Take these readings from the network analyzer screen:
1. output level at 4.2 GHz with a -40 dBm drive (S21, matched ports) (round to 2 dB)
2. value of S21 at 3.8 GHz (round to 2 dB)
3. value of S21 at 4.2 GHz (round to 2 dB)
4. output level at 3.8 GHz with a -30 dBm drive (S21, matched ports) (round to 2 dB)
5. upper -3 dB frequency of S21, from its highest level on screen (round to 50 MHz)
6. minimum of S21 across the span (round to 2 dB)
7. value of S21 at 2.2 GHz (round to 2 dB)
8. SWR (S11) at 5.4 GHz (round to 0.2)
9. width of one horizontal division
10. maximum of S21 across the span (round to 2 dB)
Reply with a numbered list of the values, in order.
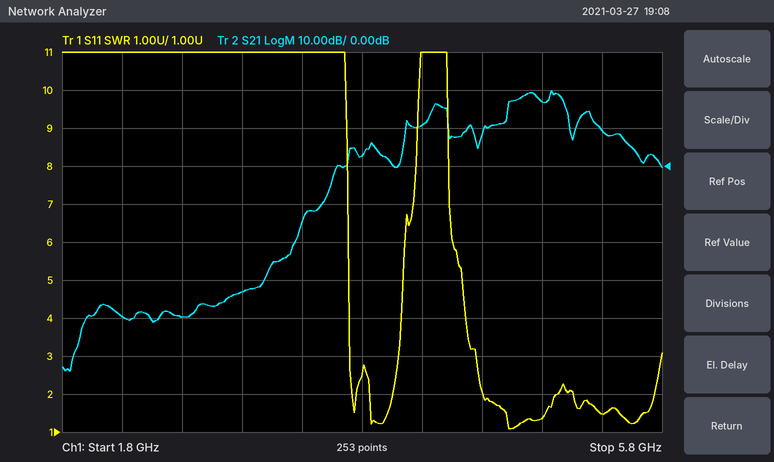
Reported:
1. -30 dBm
2. 2 dB
3. 10 dB
4. -28 dBm
5. 5.15 GHz
6. -54 dB
7. -40 dB
8. 1.4
9. 400 MHz
10. 20 dB
